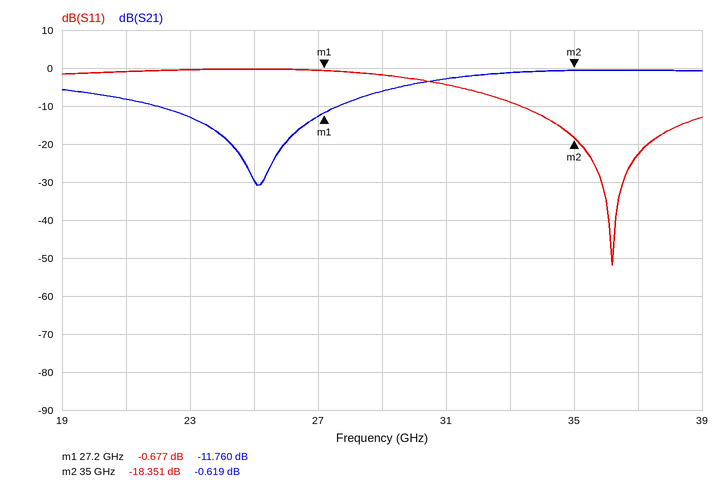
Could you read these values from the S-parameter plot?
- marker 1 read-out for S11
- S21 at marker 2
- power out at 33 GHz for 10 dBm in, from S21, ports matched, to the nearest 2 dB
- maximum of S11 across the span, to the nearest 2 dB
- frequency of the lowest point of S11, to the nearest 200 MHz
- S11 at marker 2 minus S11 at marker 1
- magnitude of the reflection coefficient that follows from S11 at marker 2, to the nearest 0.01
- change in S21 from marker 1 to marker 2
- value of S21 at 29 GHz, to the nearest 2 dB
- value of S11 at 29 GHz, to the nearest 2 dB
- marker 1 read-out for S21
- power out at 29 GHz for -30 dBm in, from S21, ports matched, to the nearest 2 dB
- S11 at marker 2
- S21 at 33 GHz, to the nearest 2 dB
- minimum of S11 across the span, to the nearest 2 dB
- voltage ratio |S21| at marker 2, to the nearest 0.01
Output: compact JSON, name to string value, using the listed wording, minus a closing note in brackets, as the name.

{"marker 1 read-out for S11": "-0.677 dB", "S21 at marker 2": "-0.619 dB", "power out at 33 GHz for 10 dBm in, from S21, ports matched, to the nearest 2 dB": "8 dBm", "maximum of S11 across the span, to the nearest 2 dB": "0 dB", "frequency of the lowest point of S11, to the nearest 200 MHz": "36.2 GHz", "S11 at marker 2 minus S11 at marker 1": "-17.674 dB", "magnitude of the reflection coefficient that follows from S11 at marker 2, to the nearest 0.01": "0.12", "change in S21 from marker 1 to marker 2": "11.141 dB", "value of S21 at 29 GHz, to the nearest 2 dB": "-6 dB", "value of S11 at 29 GHz, to the nearest 2 dB": "-2 dB", "marker 1 read-out for S21": "-11.760 dB", "power out at 29 GHz for -30 dBm in, from S21, ports matched, to the nearest 2 dB": "-36 dBm", "S11 at marker 2": "-18.351 dB", "S21 at 33 GHz, to the nearest 2 dB": "-2 dB", "minimum of S11 across the span, to the nearest 2 dB": "-52 dB", "voltage ratio |S21| at marker 2, to the nearest 0.01": "0.93"}
